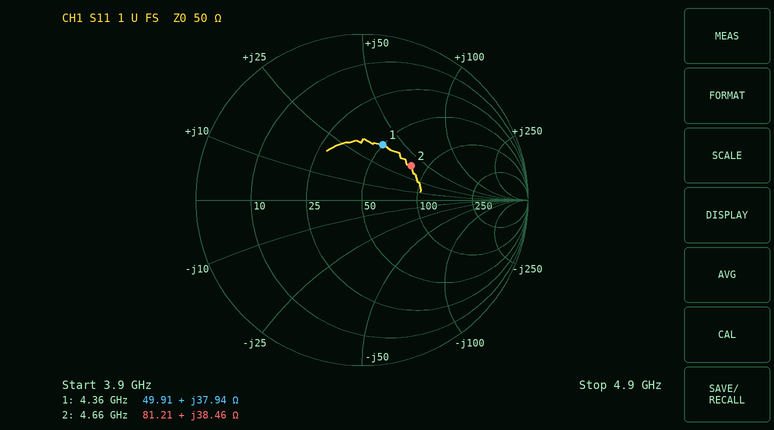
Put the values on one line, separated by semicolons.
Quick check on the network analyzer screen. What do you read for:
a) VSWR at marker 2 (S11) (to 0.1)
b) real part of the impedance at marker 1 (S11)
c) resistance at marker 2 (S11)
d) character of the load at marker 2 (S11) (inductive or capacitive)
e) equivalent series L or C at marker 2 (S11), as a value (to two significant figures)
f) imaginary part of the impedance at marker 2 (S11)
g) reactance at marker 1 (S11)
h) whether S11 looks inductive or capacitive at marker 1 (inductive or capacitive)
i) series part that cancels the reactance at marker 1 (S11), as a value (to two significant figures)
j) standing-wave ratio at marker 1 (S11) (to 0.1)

2.1; 49.91 Ω; 81.21 Ω; inductive; 1.3 nH; +38.46 Ω; +37.94 Ω; inductive; 960 fF; 2.1
